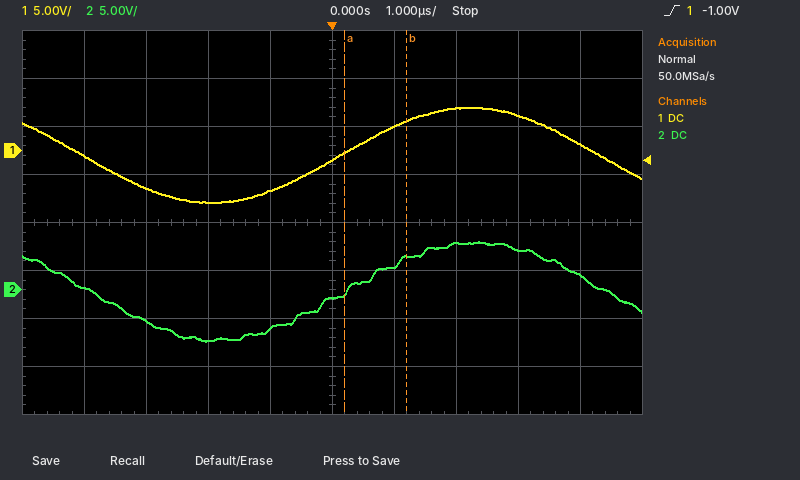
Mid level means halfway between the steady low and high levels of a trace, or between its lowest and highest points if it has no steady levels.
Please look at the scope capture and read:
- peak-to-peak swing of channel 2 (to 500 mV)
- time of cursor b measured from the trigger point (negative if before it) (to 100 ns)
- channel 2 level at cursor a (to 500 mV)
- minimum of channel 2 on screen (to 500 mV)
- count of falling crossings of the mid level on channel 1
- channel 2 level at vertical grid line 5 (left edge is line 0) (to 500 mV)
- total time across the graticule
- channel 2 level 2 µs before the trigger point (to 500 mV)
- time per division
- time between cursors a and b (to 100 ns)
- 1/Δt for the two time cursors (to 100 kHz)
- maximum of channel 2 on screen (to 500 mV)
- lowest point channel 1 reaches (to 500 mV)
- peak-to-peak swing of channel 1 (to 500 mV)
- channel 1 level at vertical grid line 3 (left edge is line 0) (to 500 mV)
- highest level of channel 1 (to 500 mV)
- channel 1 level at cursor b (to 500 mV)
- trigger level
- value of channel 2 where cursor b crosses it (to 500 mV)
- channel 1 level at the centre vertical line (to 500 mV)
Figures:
10.5 V
+1.2 µs
-500 mV
-5.5 V
2
-1.0 V
10 µs
-5.5 V
1 µs
1.0 µs
1.0 MHz
5.0 V
-5.5 V
10.0 V
-5.5 V
4.5 V
3.0 V
-1.00 V
3.5 V
-1.0 V
